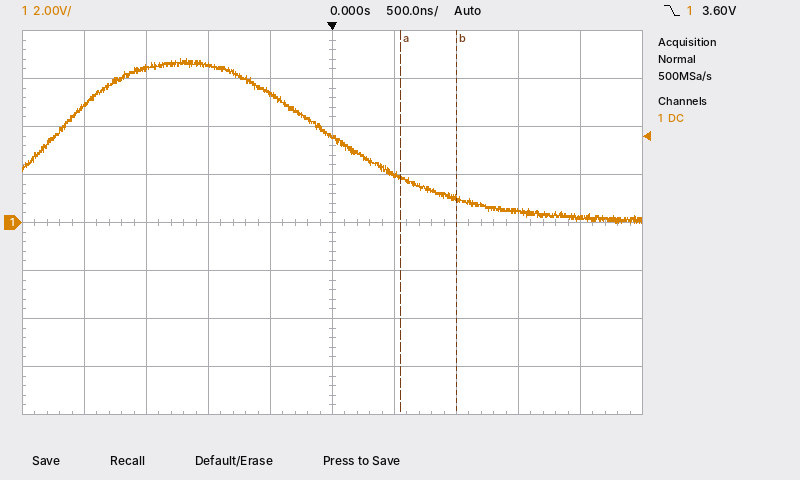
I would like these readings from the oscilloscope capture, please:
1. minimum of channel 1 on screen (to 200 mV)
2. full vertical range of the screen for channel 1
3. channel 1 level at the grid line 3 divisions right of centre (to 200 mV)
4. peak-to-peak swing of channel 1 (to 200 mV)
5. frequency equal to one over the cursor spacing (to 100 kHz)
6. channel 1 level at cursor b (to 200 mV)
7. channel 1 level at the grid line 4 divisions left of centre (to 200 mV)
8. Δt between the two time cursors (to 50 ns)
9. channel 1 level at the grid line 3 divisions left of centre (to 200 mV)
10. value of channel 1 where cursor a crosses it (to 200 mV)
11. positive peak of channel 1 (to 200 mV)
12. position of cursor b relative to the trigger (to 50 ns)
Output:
0.0 V
16 V
400 mV
6.8 V
2.2 MHz
1.0 V
4.8 V
450 ns
6.4 V
1.8 V
6.8 V
+1.00 µs
